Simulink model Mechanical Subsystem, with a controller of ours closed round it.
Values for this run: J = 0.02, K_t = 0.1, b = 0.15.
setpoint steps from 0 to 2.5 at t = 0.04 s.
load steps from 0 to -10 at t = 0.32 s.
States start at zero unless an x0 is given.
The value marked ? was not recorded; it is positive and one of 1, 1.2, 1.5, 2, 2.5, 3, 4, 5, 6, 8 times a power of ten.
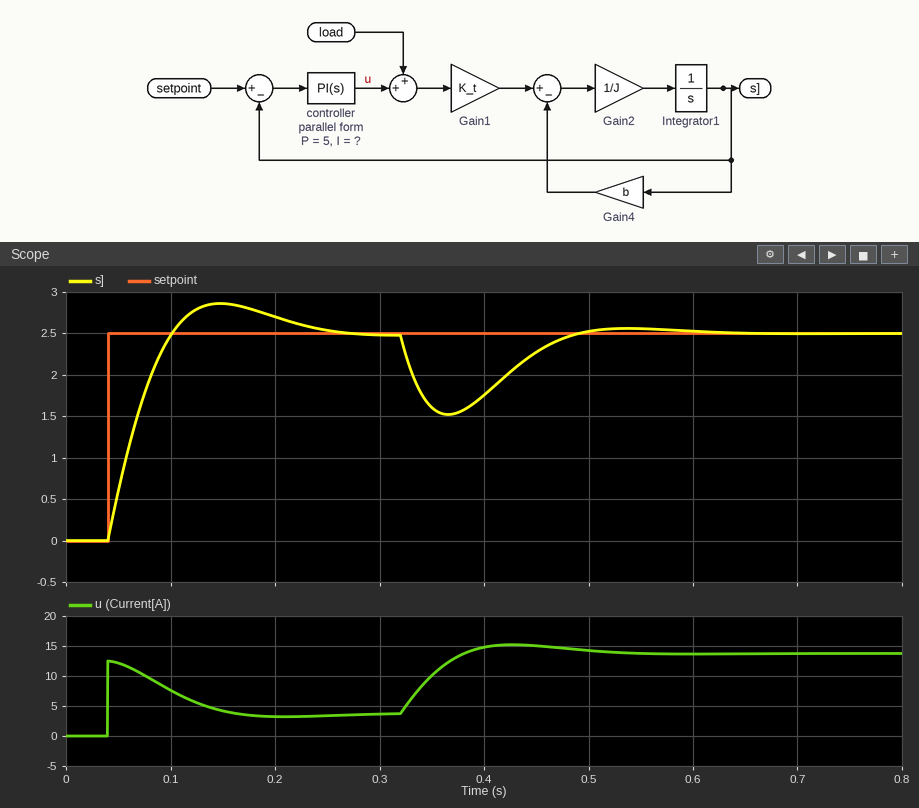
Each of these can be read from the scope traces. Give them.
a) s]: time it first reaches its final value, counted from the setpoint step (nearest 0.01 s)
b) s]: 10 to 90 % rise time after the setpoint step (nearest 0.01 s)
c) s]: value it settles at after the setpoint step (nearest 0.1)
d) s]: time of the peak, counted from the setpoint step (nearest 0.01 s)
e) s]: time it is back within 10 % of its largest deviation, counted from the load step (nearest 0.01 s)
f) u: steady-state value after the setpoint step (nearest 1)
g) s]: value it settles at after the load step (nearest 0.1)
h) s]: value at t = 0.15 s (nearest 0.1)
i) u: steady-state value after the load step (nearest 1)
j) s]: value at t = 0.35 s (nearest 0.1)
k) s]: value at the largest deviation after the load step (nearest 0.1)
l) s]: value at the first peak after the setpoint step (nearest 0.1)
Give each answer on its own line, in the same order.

0.06 s
0.05 s
2.5
0.11 s
0.15 s
4
2.5
2.9
14
1.6
1.5
2.9
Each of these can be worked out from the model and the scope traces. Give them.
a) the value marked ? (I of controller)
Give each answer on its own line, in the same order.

120
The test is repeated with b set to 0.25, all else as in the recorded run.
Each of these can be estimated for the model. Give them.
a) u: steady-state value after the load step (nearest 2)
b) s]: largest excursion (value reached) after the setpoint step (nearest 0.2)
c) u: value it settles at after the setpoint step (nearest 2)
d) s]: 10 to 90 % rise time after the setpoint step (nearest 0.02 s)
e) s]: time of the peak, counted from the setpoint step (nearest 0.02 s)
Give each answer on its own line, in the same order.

16
2.6
6
0.06 s
0.12 s
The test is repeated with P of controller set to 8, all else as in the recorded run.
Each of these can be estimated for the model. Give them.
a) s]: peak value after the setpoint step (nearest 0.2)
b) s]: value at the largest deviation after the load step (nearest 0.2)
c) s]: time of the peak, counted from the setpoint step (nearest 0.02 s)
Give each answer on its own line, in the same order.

2.6
1.8
0.10 s
